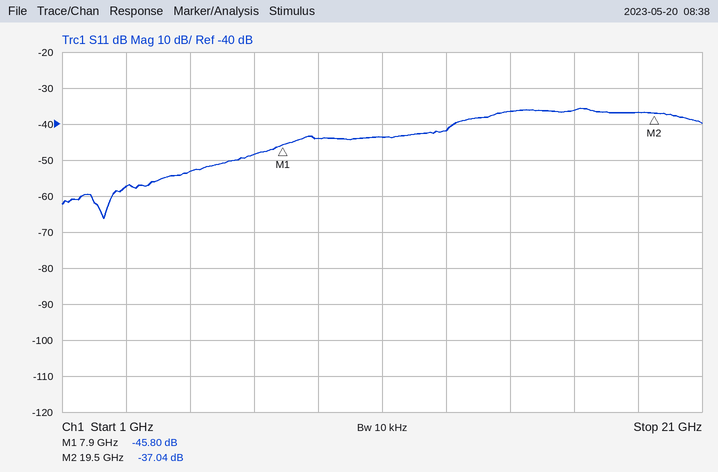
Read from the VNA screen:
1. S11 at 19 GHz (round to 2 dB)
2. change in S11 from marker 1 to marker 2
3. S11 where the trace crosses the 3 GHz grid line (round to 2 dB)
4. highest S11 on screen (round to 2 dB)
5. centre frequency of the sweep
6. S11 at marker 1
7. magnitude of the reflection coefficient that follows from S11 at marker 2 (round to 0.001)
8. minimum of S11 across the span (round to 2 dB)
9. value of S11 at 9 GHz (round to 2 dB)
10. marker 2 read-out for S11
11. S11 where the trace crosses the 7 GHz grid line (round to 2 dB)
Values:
-36 dB
8.76 dB
-58 dB
-36 dB
11 GHz
-45.80 dB
0.014
-66 dB
-44 dB
-37.04 dB
-48 dB
